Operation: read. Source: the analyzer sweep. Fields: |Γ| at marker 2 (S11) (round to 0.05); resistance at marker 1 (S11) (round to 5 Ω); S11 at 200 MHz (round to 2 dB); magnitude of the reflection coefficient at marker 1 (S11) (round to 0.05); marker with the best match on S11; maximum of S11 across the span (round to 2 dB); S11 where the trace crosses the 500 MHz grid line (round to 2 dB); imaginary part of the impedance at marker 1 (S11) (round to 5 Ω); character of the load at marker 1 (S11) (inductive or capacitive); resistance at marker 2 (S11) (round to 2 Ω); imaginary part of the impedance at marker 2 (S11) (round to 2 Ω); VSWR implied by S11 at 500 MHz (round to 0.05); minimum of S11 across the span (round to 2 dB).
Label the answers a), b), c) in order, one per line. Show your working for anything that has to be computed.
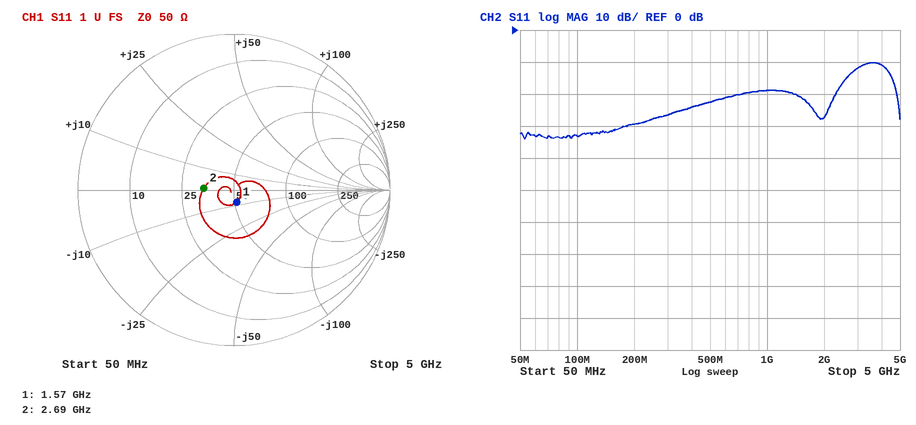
a) 0.20
b) 50 Ω
c) -30 dB
d) 0.10
e) marker 1
f) -10 dB
g) -22 dB
h) -10 Ω
i) capacitive
j) 34 Ω
k) 0 Ω
l) |Γ| = 10^(-22/20) = 0.0794; VSWR = (1 + 0.0794)/(1 − 0.0794) ≈ 1.17, so 1.15 to the nearest 0.05
m) -34 dB
